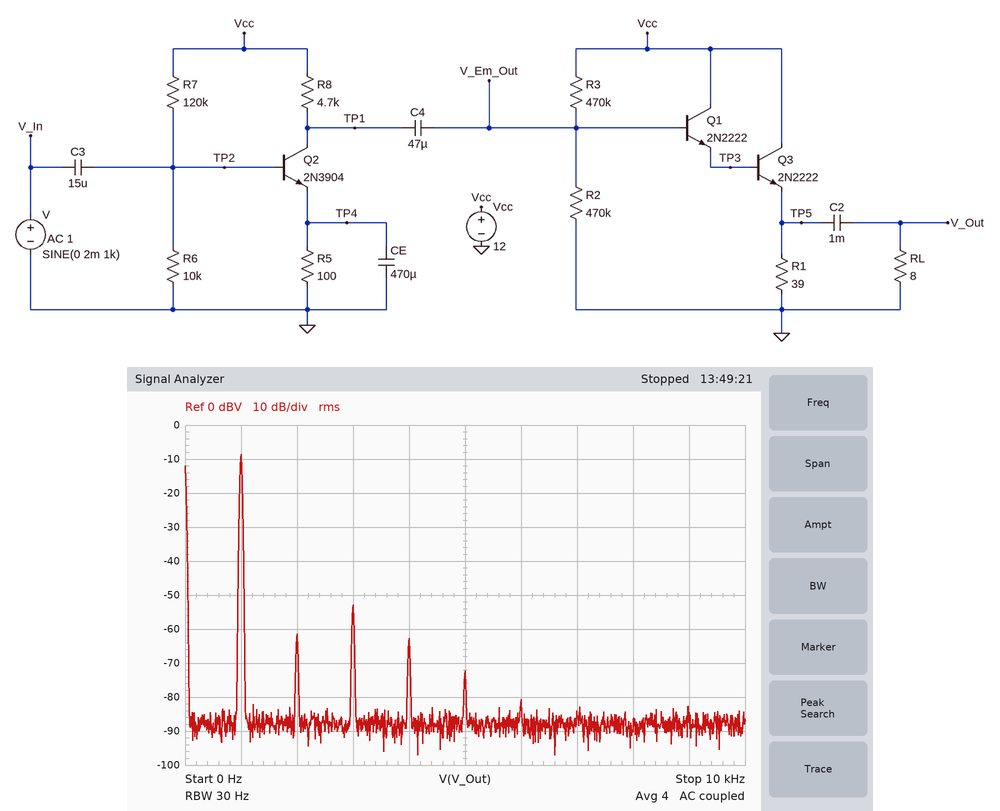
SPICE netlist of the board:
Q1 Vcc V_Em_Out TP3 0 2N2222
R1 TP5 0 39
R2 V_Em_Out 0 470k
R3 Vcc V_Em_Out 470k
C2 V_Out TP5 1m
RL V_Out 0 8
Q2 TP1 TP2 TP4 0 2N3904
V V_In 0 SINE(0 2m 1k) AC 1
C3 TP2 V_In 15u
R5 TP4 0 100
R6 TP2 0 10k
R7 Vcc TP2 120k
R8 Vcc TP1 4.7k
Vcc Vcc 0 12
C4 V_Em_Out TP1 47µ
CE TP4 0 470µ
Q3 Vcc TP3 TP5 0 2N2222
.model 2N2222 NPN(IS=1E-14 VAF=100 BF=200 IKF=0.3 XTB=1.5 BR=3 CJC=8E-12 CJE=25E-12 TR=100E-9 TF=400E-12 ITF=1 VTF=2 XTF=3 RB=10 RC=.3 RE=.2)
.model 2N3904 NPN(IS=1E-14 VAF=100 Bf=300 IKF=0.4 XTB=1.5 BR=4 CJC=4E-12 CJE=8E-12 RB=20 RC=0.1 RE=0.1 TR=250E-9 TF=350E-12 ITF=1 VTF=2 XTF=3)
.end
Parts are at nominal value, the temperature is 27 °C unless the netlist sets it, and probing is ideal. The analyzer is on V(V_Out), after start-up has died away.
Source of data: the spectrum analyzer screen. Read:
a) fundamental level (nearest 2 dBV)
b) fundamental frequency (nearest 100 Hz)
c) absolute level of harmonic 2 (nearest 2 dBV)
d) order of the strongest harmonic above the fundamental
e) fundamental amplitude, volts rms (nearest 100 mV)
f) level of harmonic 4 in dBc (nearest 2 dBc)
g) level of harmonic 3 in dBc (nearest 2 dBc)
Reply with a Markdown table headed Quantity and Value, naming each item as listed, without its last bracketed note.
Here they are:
| Quantity | Value |
|---|---|
| fundamental level | -8 dBV |
| fundamental frequency | 1.0 kHz |
| absolute level of harmonic 2 | -62 dBV |
| order of the strongest harmonic above the fundamental | 3 |
| fundamental amplitude, volts rms | 400 mV |
| level of harmonic 4 in dBc | -54 dBc |
| level of harmonic 3 in dBc | -44 dBc |
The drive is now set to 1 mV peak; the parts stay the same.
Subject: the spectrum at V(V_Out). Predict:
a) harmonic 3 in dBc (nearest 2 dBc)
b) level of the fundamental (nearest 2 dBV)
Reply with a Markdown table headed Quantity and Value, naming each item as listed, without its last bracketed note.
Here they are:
| Quantity | Value |
|---|---|
| harmonic 3 in dBc | -60 dBc |
| level of the fundamental | -14 dBV |
